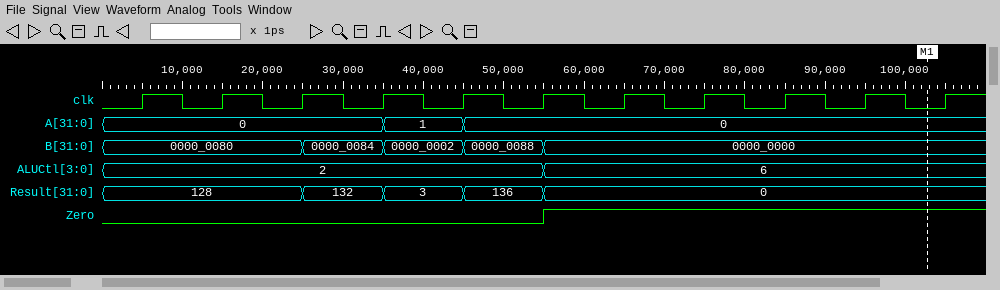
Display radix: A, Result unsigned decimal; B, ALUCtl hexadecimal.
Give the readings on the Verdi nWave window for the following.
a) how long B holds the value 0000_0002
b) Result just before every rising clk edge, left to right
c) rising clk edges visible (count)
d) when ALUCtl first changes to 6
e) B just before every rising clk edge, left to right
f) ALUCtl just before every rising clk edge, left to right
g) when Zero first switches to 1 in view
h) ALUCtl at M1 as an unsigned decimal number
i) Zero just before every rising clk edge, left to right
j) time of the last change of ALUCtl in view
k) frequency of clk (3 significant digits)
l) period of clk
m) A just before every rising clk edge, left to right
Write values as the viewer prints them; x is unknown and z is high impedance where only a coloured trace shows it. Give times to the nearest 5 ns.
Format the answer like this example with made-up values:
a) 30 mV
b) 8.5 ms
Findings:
a) 10 ns
b) 128, 128, 128, 132, 3, 136, 0, 0, 0, 0, 0
c) 11
d) 55 ns
e) 0000_0080, 0000_0080, 0000_0080, 0000_0084, 0000_0002, 0000_0088, 0000_0000, 0000_0000, 0000_0000, 0000_0000, 0000_0000
f) 2, 2, 2, 2, 2, 2, 6, 6, 6, 6, 6
g) 55 ns
h) 6
i) 0 0 0 0 0 0 1 1 1 1 1
j) 55 ns
k) 100 MHz
l) 10 ns
m) 0, 0, 0, 0, 1, 0, 0, 0, 0, 0, 0
